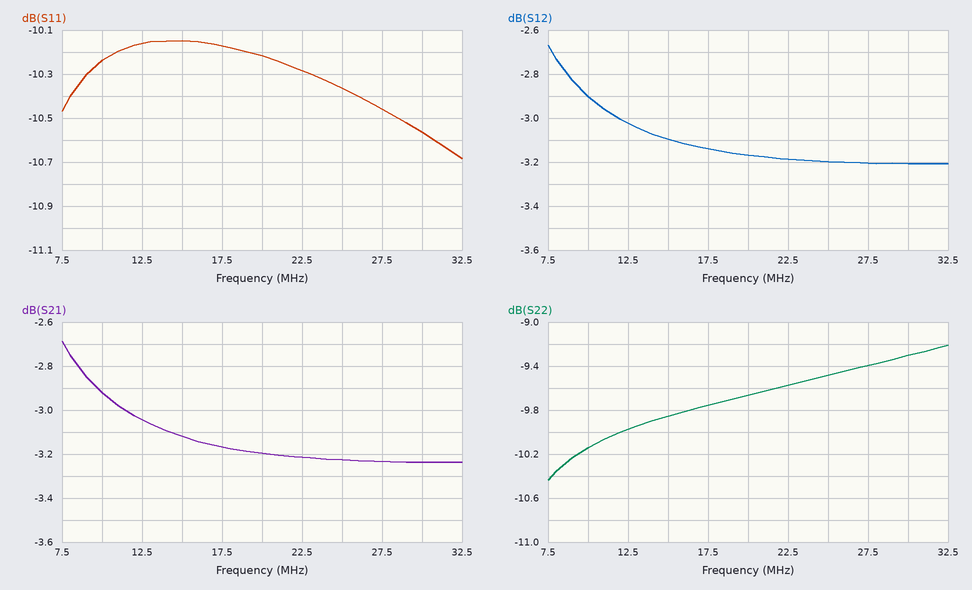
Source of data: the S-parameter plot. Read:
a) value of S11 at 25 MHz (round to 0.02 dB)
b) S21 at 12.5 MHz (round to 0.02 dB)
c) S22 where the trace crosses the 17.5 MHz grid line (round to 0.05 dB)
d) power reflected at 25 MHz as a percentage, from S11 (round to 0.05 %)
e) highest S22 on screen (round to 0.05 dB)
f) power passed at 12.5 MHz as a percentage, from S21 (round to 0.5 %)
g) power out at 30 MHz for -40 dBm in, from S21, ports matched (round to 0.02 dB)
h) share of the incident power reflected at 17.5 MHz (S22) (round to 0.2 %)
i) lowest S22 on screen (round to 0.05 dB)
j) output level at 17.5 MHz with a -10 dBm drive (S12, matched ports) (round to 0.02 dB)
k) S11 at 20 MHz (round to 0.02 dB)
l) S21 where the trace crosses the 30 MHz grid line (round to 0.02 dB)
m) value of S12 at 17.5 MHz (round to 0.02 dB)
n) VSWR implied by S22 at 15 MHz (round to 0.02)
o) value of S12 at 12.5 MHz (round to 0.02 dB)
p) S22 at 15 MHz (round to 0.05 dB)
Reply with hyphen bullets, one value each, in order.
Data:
- -10.36 dB
- -3.04 dB
- -9.75 dB
- 9.20 %
- -9.20 dB
- 49.5 %
- -43.24 dBm
- 10.6 %
- -10.45 dB
- -13.14 dBm
- -10.22 dB
- -3.24 dB
- -3.14 dB
- 1.94
- -3.02 dB
- -9.85 dB
